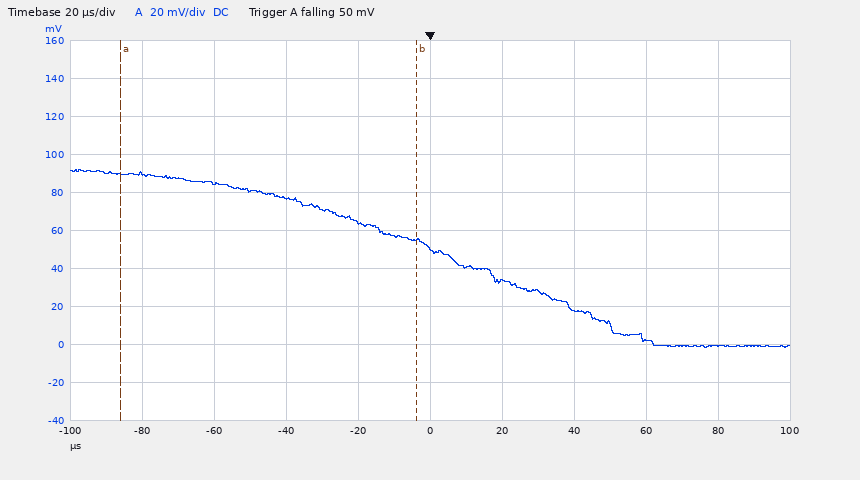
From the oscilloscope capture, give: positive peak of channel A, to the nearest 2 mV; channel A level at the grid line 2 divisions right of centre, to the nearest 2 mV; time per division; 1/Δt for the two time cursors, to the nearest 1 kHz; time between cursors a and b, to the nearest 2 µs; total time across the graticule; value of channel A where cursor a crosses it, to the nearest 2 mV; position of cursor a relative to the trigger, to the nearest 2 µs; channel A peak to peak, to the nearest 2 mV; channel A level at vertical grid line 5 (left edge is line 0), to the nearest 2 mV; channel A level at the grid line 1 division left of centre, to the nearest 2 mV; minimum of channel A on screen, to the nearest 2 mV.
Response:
92 mV
18 mV
20 µs
12 kHz
82 µs
200 µs
90 mV
-86 µs
94 mV
50 mV
64 mV
-2 mV
